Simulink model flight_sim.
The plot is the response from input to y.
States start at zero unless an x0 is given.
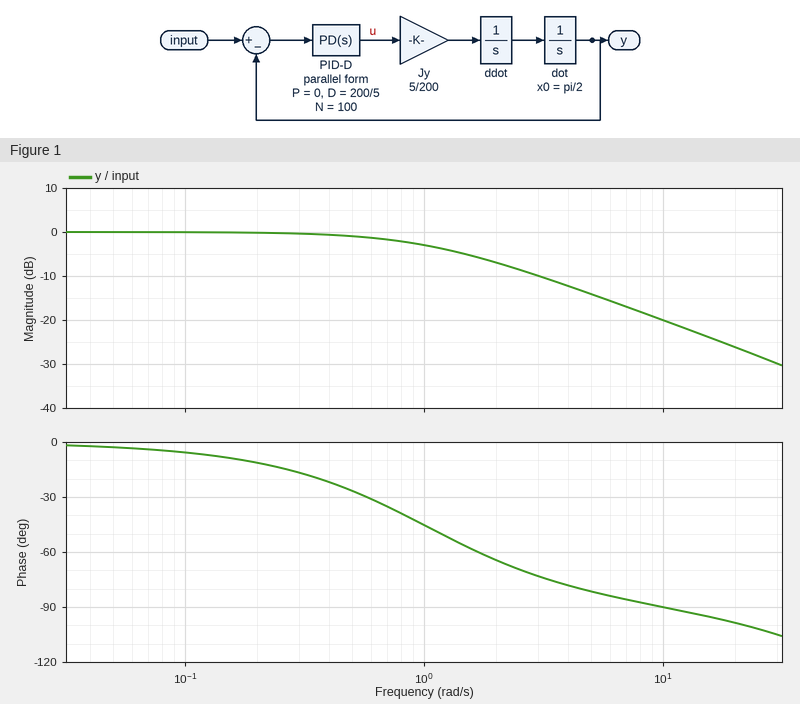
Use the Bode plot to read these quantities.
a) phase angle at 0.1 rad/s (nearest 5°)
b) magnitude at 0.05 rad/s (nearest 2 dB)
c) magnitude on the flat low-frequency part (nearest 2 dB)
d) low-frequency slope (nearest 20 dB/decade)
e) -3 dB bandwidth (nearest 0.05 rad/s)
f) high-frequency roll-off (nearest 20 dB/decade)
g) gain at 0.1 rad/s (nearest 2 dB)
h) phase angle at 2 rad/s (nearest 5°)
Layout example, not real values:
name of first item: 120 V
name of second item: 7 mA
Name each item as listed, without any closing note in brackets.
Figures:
phase angle at 0.1 rad/s: -5°
magnitude at 0.05 rad/s: 0 dB
magnitude on the flat low-frequency part: 0 dB
low-frequency slope: 0 dB/decade
-3 dB bandwidth: 1.00 rad/s
high-frequency roll-off: -20 dB/decade
gain at 0.1 rad/s: 0 dB
phase angle at 2 rad/s: -65°
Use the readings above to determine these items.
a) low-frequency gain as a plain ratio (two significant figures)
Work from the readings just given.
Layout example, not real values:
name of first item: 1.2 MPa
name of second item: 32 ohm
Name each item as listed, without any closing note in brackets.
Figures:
low-frequency gain as a plain ratio: 1.0
